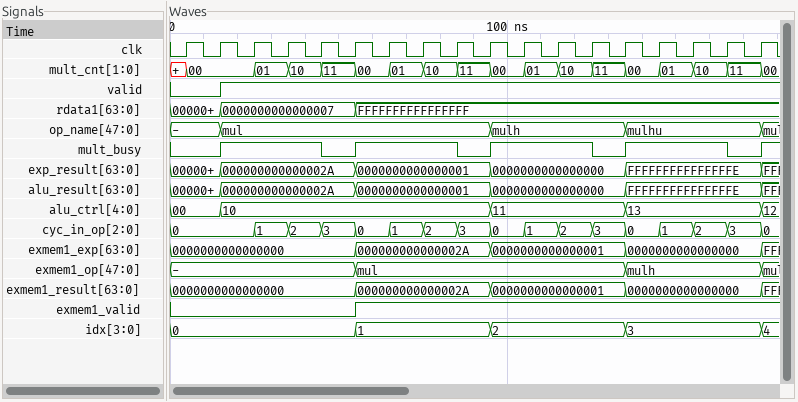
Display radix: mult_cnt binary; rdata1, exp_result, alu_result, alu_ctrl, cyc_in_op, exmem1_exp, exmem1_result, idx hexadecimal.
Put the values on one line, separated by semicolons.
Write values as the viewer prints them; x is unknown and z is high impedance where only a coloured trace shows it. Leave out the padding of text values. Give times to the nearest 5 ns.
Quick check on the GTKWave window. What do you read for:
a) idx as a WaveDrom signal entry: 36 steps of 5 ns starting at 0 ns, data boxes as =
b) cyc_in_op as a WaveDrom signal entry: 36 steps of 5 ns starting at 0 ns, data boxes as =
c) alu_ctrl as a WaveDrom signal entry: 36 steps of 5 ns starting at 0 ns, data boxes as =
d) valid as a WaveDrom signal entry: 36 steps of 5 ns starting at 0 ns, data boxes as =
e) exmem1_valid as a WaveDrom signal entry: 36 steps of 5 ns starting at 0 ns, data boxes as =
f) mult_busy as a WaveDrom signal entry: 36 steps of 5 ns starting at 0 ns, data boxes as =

{name: 'idx', wave: '=..........=.......=.......=.......=', data: '0 1 2 3 4'}; {name: 'cyc_in_op', wave: '=....=.=.=.=.=.=.=.=.=.=.=.=.=.=.=.=', data: '0 1 2 3 0 1 2 3 0 1 2 3 0 1 2 3 0'}; {name: 'alu_ctrl', wave: '=..=...............=.......=.......=', data: '00 10 11 13 12'}; {name: 'valid', wave: '0..1................................'}; {name: 'exmem1_valid', wave: '0..........1........................'}; {name: 'mult_busy', wave: '0..1.....0.1.....0.1.....0.1.....0.1'}
